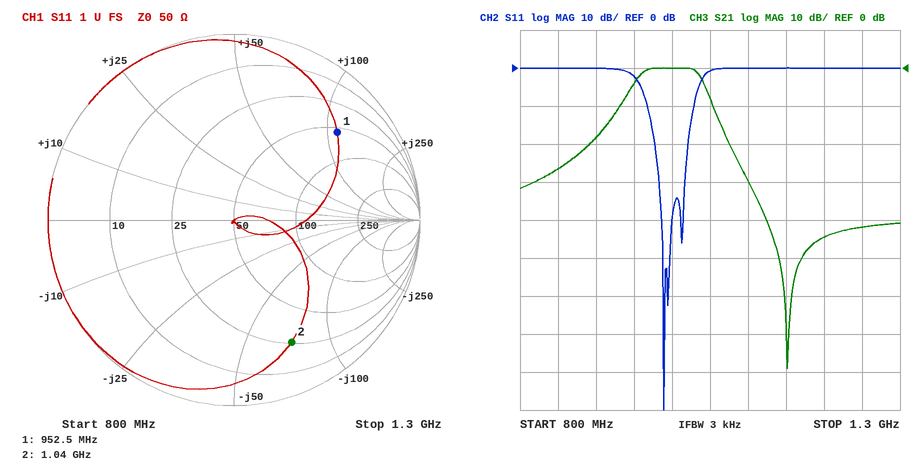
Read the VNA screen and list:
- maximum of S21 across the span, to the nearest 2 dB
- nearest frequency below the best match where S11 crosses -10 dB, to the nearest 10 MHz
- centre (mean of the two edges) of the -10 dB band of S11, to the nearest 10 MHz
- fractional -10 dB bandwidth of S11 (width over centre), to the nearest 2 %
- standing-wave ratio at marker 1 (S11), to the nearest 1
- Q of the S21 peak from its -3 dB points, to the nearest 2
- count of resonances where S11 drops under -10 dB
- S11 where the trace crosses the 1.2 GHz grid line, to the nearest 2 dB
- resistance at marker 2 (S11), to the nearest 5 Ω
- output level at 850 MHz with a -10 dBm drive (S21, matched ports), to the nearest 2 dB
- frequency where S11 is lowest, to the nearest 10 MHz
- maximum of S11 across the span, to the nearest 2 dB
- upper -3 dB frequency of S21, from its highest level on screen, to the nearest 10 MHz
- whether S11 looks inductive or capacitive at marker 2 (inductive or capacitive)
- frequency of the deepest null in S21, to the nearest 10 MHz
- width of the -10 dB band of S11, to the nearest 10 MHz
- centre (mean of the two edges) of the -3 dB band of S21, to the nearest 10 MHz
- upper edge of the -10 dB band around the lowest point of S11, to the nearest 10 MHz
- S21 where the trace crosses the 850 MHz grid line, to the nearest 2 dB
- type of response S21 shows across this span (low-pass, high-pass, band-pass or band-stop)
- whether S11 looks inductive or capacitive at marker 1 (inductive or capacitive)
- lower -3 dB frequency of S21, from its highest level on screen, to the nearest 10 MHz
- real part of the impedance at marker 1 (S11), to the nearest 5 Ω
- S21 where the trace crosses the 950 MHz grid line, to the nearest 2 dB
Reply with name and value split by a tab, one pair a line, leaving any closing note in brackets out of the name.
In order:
maximum of S21 across the span, to the nearest 2 dB	0 dB
nearest frequency below the best match where S11 crosses -10 dB, to the nearest 10 MHz	970 MHz
centre (mean of the two edges) of the -10 dB band of S11, to the nearest 10 MHz	1.00 GHz
fractional -10 dB bandwidth of S11 (width over centre), to the nearest 2 %	6 %
standing-wave ratio at marker 1 (S11), to the nearest 1	6
Q of the S21 peak from its -3 dB points, to the nearest 2	12
count of resonances where S11 drops under -10 dB	3
S11 where the trace crosses the 1.2 GHz grid line, to the nearest 2 dB	0 dB
resistance at marker 2 (S11), to the nearest 5 Ω	25 Ω
output level at 850 MHz with a -10 dBm drive (S21, matched ports), to the nearest 2 dB	-36 dBm
frequency where S11 is lowest, to the nearest 10 MHz	990 MHz
maximum of S11 across the span, to the nearest 2 dB	0 dB
upper -3 dB frequency of S21, from its highest level on screen, to the nearest 10 MHz	1.04 GHz
whether S11 looks inductive or capacitive at marker 2	capacitive
frequency of the deepest null in S21, to the nearest 10 MHz	1.15 GHz
width of the -10 dB band of S11, to the nearest 10 MHz	60 MHz
centre (mean of the two edges) of the -3 dB band of S21, to the nearest 10 MHz	1.00 GHz
upper edge of the -10 dB band around the lowest point of S11, to the nearest 10 MHz	1.03 GHz
S21 where the trace crosses the 850 MHz grid line, to the nearest 2 dB	-26 dB
type of response S21 shows across this span	band-pass
whether S11 looks inductive or capacitive at marker 1	inductive
lower -3 dB frequency of S21, from its highest level on screen, to the nearest 10 MHz	950 MHz
real part of the impedance at marker 1 (S11), to the nearest 5 Ω	55 Ω
S21 where the trace crosses the 950 MHz grid line, to the nearest 2 dB	-4 dB
